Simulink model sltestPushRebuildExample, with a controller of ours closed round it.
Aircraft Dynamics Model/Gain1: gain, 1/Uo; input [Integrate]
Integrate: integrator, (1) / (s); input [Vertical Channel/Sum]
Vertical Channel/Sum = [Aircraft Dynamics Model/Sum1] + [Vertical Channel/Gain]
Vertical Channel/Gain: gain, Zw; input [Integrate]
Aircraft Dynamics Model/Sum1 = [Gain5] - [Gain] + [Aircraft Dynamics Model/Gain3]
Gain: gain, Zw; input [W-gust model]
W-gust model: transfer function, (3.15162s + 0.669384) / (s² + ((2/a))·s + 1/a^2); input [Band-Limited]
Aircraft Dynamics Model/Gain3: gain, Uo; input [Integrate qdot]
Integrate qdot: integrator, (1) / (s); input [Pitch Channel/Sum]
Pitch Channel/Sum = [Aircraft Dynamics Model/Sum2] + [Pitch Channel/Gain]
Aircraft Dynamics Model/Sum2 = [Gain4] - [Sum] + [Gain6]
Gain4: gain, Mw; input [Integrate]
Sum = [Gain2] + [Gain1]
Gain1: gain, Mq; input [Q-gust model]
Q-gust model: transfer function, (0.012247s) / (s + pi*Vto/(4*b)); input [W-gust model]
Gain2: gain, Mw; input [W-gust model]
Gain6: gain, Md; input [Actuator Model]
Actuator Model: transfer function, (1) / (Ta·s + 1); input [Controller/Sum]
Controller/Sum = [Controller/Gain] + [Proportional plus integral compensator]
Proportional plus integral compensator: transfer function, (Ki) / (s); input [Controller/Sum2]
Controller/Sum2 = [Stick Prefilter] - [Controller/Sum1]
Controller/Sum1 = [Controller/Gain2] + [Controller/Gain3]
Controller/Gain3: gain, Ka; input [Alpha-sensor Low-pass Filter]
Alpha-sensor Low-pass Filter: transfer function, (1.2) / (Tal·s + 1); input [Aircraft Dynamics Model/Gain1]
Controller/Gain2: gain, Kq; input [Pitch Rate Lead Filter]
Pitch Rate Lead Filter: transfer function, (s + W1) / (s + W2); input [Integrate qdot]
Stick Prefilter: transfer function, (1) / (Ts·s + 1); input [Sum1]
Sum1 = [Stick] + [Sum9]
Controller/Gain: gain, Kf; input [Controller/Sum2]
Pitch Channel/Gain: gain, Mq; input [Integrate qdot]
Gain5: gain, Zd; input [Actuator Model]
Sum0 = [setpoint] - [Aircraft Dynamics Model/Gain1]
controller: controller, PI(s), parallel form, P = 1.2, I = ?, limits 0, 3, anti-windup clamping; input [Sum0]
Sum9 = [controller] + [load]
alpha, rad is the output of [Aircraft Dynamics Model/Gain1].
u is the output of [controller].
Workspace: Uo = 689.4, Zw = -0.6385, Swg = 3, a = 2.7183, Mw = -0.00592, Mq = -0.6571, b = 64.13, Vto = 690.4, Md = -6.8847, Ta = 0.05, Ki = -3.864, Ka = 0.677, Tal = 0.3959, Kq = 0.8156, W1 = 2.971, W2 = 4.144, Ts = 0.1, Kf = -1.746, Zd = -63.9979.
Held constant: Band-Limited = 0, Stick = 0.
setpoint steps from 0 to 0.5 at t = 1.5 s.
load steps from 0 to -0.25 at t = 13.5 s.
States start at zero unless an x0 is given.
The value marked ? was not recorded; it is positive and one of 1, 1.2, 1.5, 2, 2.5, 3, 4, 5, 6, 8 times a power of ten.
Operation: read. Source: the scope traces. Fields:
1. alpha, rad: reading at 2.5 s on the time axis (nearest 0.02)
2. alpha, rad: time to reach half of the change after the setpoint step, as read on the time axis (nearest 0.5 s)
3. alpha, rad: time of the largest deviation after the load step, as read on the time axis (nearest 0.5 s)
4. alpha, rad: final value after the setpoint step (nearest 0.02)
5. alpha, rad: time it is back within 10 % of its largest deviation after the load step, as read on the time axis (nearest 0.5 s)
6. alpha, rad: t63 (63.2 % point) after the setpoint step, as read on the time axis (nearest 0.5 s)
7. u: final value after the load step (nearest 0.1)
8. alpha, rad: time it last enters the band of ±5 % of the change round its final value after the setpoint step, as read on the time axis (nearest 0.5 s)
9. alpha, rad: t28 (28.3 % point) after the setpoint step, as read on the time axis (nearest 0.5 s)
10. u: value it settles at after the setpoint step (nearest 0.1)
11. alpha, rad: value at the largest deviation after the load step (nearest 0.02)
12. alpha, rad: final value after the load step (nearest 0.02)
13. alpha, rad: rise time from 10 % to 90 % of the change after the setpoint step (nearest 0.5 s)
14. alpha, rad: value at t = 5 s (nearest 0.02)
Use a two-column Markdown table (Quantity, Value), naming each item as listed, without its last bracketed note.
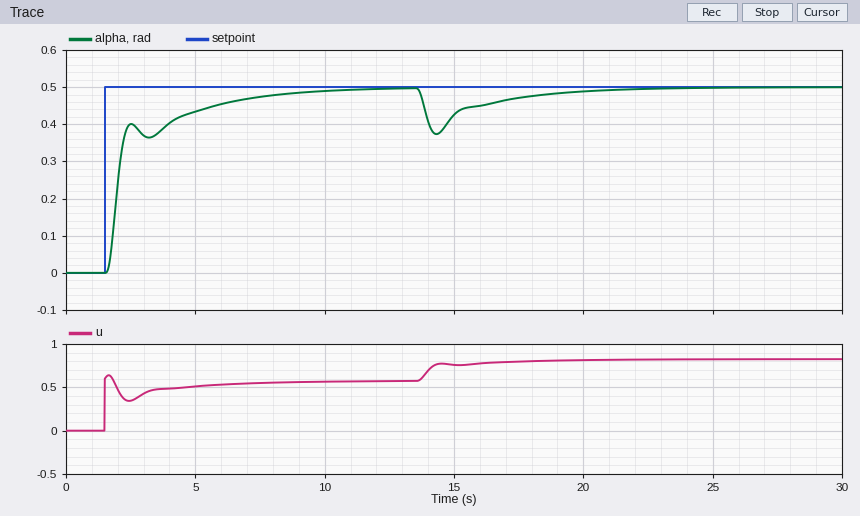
| Quantity | Value |
|---|---|
| alpha, rad: reading at 2.5 s on the time axis | 0.40 |
| alpha, rad: time to reach half of the change after the setpoint step, as read on the time axis | 2.0 s |
| alpha, rad: time of the largest deviation after the load step, as read on the time axis | 14.5 s |
| alpha, rad: final value after the setpoint step | 0.50 |
| alpha, rad: time it is back within 10 % of its largest deviation after the load step, as read on the time axis | 20.0 s |
| alpha, rad: t63 (63.2 % point) after the setpoint step, as read on the time axis | 2.0 s |
| u: final value after the load step | 0.8 |
| alpha, rad: time it last enters the band of ±5 % of the change round its final value after the setpoint step, as read on the time axis | 7.5 s |
| alpha, rad: t28 (28.3 % point) after the setpoint step, as read on the time axis | 2.0 s |
| u: value it settles at after the setpoint step | 0.6 |
| alpha, rad: value at the largest deviation after the load step | 0.38 |
| alpha, rad: final value after the load step | 0.50 |
| alpha, rad: rise time from 10 % to 90 % of the change after the setpoint step | 4.0 s |
| alpha, rad: value at t = 5 s | 0.44 |
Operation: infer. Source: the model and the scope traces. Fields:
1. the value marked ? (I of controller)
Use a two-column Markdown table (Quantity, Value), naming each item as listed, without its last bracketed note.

| Quantity | Value |
|---|---|
| the value marked ? | 0.8 |
